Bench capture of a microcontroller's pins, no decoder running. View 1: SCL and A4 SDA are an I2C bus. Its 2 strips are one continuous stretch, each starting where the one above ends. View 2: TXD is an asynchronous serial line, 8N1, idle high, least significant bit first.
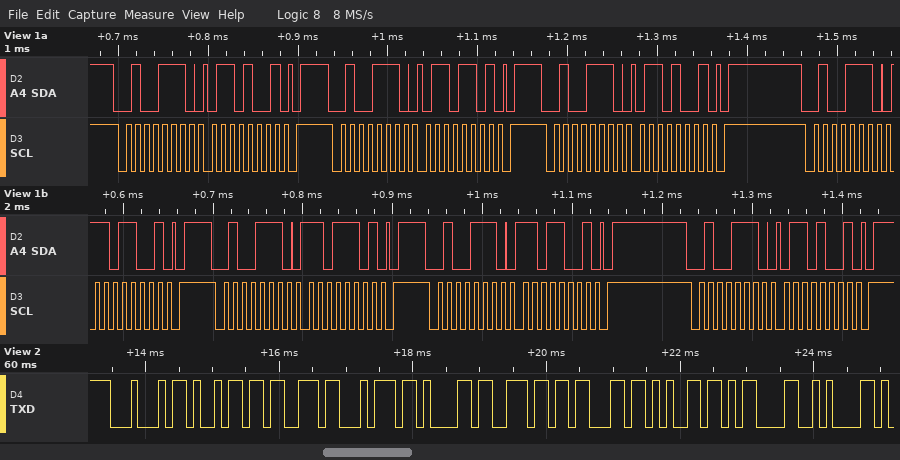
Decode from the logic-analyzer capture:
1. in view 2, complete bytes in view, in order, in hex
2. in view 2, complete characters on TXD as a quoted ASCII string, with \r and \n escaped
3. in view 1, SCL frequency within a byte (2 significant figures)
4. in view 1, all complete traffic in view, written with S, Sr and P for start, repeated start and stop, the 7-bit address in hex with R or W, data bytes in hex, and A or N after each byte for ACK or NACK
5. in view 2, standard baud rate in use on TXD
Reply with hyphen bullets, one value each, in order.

- 0x44 0x69 0x73 0x74 0x61 0x6E 0x63 0x65 0x0D 0x0A
- "Distance\r\n"
- 100 kHz
- S 27W A 69 A P S 27W A 6D A P S 27W A 69 A P S 27W A D9 A P S 27W A DD A P S 27W A D9 A P S 27W A 69 A P
- 9600 baud
